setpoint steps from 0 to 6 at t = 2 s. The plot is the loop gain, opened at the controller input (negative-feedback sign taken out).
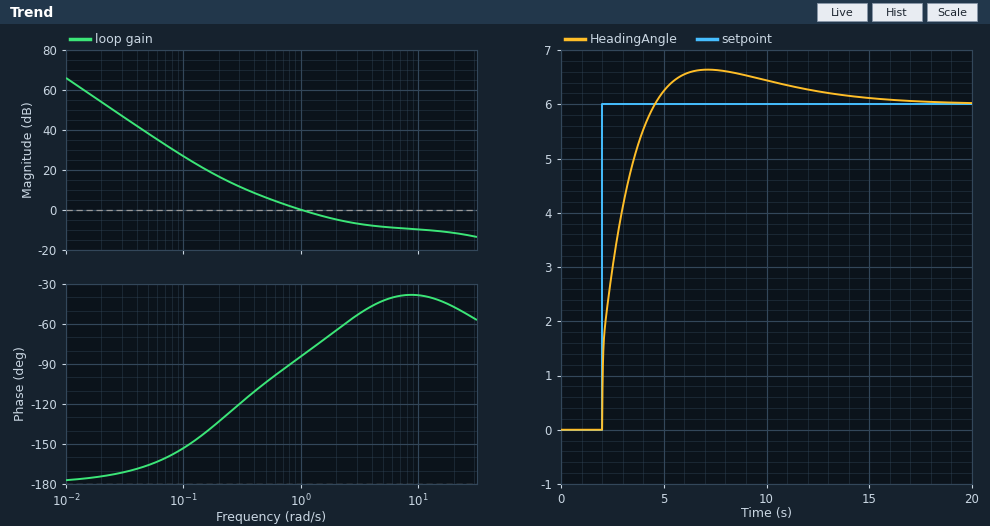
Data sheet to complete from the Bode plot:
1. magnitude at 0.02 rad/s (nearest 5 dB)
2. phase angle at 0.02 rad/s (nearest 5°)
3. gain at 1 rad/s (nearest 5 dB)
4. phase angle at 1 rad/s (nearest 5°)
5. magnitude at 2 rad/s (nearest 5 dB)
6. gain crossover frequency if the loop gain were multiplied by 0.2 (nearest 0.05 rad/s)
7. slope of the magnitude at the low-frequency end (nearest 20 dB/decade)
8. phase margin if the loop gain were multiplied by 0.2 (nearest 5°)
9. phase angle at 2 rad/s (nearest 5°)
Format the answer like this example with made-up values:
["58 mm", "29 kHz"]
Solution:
["55 dB", "-175°", "0 dB", "-85°", "-5 dB", "0.25 rad/s", "-40 dB/decade", "55°", "-65°"]
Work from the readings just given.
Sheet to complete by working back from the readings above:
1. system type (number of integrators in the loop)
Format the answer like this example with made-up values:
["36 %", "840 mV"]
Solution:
["2"]
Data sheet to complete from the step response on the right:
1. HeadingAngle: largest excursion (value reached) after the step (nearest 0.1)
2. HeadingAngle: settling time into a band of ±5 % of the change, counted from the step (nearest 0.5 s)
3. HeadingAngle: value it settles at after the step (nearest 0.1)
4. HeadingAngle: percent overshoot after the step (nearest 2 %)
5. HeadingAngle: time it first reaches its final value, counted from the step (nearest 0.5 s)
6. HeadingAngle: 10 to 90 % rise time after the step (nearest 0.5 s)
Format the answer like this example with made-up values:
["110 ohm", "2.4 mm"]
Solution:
["6.6", "9.5 s", "6.0", "10 %", "2.5 s", "2.0 s"]
